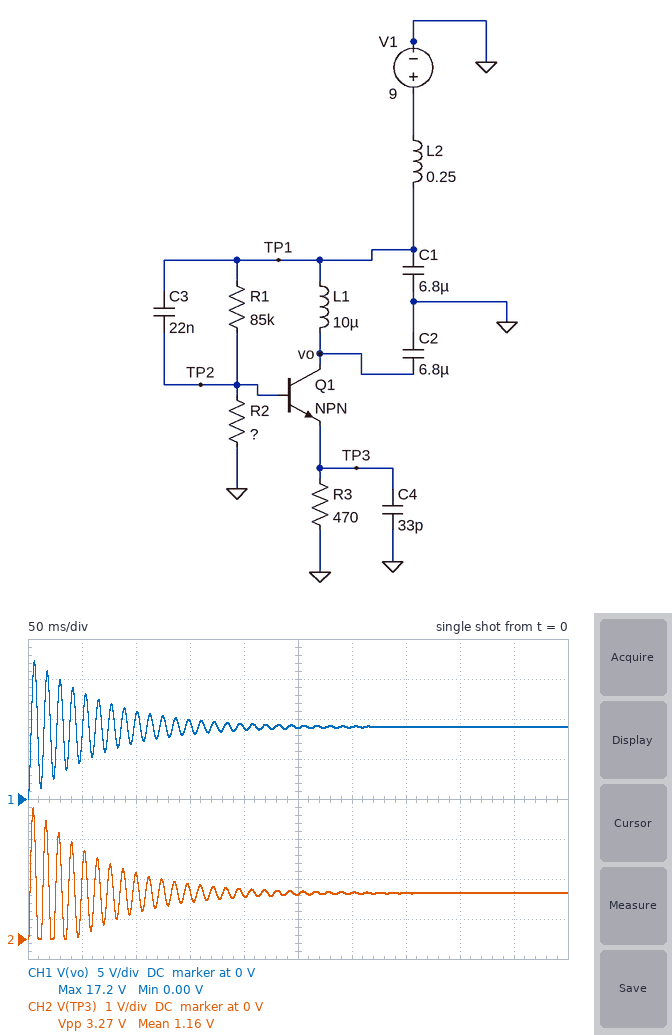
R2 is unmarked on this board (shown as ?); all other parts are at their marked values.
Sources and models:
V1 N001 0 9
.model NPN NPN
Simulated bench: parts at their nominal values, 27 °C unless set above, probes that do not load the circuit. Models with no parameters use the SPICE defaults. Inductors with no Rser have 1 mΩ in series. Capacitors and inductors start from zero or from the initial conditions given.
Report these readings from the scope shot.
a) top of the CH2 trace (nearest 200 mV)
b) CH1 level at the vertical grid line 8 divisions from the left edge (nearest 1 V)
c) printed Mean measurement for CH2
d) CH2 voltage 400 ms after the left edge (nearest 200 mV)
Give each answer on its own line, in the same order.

3.2 V
9 V
1.16 V
1.2 V
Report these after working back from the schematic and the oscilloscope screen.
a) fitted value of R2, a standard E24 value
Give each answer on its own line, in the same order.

33 kΩ
